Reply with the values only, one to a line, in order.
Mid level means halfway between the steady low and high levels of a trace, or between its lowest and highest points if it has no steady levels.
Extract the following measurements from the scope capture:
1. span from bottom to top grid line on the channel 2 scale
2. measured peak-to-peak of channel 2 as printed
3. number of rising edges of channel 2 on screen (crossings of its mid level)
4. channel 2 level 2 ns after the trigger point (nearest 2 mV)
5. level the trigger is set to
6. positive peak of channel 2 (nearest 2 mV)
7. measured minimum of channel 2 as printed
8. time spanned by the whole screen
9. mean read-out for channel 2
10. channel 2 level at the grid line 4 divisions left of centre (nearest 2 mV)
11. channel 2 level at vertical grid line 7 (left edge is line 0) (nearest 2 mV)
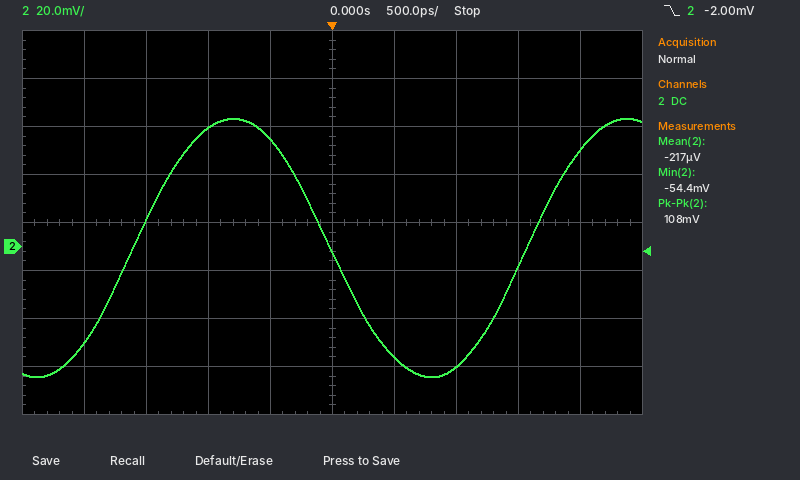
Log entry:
160 mV
108 mV
2
40 mV
-2.00 mV
54 mV
-54.4 mV
5 ns
-217 µV
-40 mV
-50 mV
